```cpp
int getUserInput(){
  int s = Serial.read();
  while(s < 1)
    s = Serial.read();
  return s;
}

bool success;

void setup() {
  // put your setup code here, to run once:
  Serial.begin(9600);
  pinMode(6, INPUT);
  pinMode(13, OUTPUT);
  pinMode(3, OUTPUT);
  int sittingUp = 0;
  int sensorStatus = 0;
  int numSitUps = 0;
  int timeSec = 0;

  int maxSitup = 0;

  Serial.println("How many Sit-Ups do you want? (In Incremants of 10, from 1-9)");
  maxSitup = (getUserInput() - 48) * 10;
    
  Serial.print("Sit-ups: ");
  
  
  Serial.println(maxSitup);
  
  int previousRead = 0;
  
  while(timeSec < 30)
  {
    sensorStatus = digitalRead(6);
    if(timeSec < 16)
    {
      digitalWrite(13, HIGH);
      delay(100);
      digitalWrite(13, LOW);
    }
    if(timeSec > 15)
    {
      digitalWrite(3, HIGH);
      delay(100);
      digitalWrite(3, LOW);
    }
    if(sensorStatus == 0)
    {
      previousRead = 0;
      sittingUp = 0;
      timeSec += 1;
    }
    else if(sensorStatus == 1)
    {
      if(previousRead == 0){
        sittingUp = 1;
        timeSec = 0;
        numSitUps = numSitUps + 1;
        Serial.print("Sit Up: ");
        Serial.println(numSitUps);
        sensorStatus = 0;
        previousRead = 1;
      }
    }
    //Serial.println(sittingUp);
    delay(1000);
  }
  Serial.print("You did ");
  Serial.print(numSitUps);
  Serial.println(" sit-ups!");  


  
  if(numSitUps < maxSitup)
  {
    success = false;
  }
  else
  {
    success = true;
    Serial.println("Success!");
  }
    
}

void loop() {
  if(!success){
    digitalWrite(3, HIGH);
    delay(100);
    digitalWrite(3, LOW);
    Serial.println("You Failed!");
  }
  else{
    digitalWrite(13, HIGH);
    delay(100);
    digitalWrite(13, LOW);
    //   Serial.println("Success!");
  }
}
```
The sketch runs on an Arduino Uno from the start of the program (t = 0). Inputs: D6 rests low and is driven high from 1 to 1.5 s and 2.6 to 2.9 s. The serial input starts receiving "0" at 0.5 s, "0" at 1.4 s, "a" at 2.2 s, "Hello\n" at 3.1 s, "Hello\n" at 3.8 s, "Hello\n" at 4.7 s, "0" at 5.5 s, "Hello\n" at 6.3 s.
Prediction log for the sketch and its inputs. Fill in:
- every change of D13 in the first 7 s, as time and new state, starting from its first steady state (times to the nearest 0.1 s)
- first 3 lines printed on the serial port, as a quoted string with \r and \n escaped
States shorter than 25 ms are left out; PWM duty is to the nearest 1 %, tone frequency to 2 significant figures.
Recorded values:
0 s low; 0.5 s high; 0.6 s low; 1.6 s high; 1.7 s low; 2.7 s high; 2.8 s low; 3.8 s high; 3.9 s low; 4.9 s high; 5 s low; 6 s high; 6.1 s low
"How many Sit-Ups do you want? (In Incremants of 10, from 1-9)\r\nSit-ups: 0\r\nSit Up: 1\r\n"
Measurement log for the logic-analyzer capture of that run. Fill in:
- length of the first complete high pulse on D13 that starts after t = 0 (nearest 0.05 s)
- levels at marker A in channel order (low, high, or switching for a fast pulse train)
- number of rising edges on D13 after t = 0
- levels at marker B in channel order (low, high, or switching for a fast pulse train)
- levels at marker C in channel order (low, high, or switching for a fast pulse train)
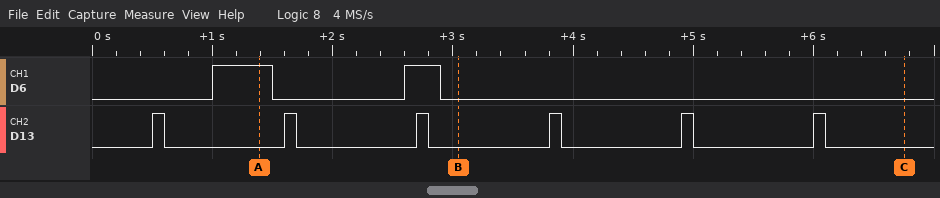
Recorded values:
0.10 s
D6 high, D13 low
6
D6 low, D13 low
D6 low, D13 low
